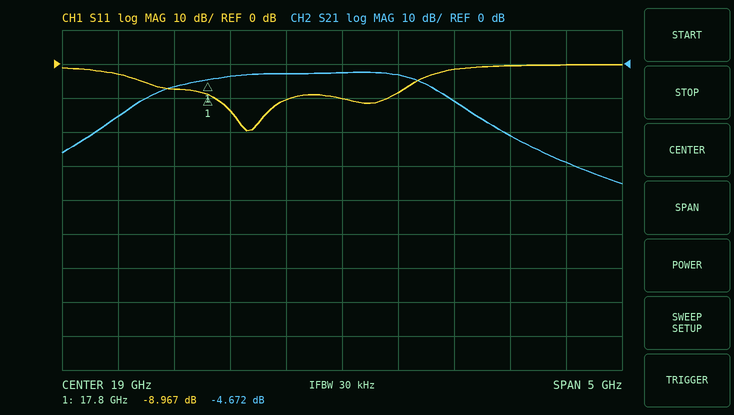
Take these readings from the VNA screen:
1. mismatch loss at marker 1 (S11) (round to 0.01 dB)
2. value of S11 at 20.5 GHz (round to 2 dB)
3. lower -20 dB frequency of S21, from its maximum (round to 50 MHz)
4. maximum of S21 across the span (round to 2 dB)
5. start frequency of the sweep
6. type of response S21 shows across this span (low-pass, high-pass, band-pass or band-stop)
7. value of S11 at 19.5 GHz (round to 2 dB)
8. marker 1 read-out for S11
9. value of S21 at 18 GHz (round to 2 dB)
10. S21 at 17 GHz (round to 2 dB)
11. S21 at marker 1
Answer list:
0.59 dB
0 dB
16.70 GHz
-2 dB
16.5 GHz
band-pass
-8 dB
-8.967 dB
-4 dB
-16 dB
-4.672 dB
